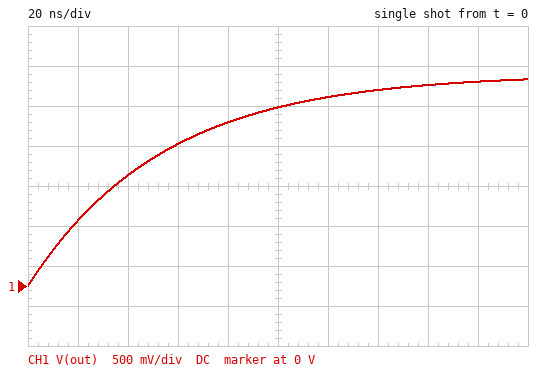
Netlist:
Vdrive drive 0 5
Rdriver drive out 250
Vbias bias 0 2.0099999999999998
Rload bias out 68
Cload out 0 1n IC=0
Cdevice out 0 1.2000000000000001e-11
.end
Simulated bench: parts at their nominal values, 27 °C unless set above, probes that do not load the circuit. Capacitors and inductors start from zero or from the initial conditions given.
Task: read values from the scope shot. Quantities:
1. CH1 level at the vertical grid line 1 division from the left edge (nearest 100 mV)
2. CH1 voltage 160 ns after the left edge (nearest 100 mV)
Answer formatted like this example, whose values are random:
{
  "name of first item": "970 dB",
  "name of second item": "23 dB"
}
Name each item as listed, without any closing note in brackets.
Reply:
{
  "CH1 level at the vertical grid line 1 division from the left edge": "800 mV",
  "CH1 voltage 160 ns after the left edge": "2.5 V"
}
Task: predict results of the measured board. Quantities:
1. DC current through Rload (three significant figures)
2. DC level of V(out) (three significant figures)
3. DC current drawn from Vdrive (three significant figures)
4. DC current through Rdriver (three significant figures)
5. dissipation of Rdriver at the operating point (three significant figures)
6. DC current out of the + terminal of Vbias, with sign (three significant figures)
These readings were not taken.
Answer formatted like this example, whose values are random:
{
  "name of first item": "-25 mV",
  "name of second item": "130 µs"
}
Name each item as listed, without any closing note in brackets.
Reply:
{
  "DC current through Rload": "9.40 mA",
  "DC level of V(out)": "2.65 V",
  "DC current drawn from Vdrive": "9.40 mA",
  "DC current through Rdriver": "9.40 mA",
  "dissipation of Rdriver at the operating point": "22.1 mW",
  "DC current out of the + terminal of Vbias, with sign": "-9.40 mA"
}
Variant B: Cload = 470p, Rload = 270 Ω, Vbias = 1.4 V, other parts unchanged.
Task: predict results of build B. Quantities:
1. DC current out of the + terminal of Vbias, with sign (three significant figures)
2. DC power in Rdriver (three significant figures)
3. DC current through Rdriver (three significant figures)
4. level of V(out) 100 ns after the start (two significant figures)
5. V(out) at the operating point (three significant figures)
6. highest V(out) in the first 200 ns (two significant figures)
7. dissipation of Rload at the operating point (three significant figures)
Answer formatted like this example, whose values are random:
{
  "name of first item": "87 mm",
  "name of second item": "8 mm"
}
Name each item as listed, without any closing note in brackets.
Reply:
{
  "DC current out of the + terminal of Vbias, with sign": "-6.92 mA",
  "DC power in Rdriver": "12.0 mW",
  "DC current through Rdriver": "6.92 mA",
  "level of V(out) 100 ns after the start": "2.6 V",
  "V(out) at the operating point": "3.27 V",
  "highest V(out) in the first 200 ns": "3.1 V",
  "dissipation of Rload at the operating point": "12.9 mW"
}
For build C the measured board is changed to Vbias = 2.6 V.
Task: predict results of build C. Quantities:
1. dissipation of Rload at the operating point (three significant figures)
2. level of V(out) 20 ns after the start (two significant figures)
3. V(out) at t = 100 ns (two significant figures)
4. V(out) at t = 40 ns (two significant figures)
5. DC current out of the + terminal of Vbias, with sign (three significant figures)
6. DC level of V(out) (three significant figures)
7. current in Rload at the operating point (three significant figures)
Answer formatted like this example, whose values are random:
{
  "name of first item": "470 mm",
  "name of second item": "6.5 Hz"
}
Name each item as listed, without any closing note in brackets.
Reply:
{
  "dissipation of Rload at the operating point": "3.87 mW",
  "level of V(out) 20 ns after the start": "960 mV",
  "V(out) at t = 100 ns": "2.6 V",
  "V(out) at t = 40 ns": "1.6 V",
  "DC current out of the + terminal of Vbias, with sign": "-7.55 mA",
  "DC level of V(out)": "3.11 V",
  "current in Rload at the operating point": "7.55 mA"
}
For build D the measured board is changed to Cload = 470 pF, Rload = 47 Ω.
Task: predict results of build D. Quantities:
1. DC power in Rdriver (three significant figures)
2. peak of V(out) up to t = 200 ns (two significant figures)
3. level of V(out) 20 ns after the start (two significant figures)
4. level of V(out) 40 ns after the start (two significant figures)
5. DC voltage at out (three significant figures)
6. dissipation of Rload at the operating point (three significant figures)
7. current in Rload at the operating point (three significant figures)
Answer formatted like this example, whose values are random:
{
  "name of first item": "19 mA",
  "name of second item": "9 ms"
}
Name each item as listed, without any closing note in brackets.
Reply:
{
  "DC power in Rdriver": "25.3 mW",
  "peak of V(out) up to t = 200 ns": "2.5 V",
  "level of V(out) 20 ns after the start": "1.6 V",
  "level of V(out) 40 ns after the start": "2.2 V",
  "DC voltage at out": "2.48 V",
  "dissipation of Rload at the operating point": "4.76 mW",
  "current in Rload at the operating point": "10.1 mA"
}
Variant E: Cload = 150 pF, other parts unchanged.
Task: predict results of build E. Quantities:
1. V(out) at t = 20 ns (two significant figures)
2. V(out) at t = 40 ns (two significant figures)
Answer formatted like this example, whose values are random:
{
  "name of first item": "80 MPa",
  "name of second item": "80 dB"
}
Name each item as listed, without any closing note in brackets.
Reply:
{
  "V(out) at t = 20 ns": "2.4 V",
  "V(out) at t = 40 ns": "2.6 V"
}
